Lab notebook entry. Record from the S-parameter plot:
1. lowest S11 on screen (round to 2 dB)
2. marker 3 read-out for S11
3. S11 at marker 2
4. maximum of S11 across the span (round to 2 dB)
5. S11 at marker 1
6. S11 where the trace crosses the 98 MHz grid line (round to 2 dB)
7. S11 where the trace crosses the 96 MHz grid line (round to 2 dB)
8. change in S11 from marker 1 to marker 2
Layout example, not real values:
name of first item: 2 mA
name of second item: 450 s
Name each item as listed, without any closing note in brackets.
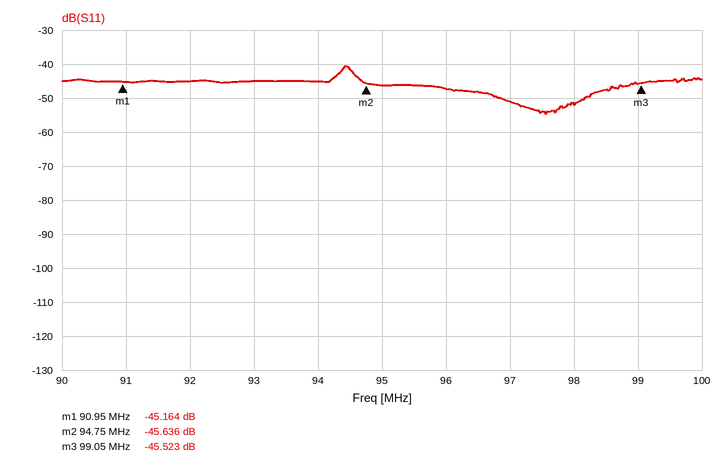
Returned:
lowest S11 on screen: -54 dB
marker 3 read-out for S11: -45.523 dB
S11 at marker 2: -45.636 dB
maximum of S11 across the span: -40 dB
S11 at marker 1: -45.164 dB
S11 where the trace crosses the 98 MHz grid line: -52 dB
S11 where the trace crosses the 96 MHz grid line: -48 dB
change in S11 from marker 1 to marker 2: -0.472 dB
